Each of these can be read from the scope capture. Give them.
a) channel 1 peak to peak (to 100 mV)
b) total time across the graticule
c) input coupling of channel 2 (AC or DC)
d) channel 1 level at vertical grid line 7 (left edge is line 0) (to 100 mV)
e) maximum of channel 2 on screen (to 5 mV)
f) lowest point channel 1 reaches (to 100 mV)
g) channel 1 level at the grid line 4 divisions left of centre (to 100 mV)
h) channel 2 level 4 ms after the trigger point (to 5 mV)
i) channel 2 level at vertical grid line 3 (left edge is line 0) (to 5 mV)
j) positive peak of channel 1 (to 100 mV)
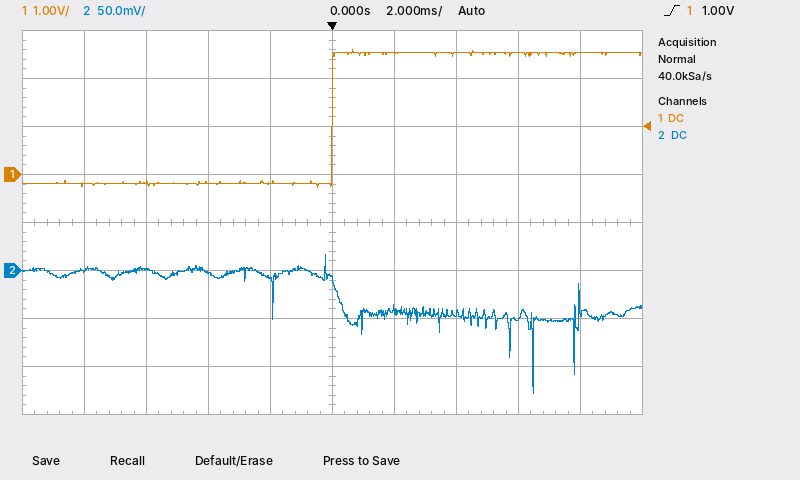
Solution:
2.9 V
20 ms
DC
2.5 V
15 mV
-300 mV
-200 mV
-45 mV
-5 mV
2.6 V
